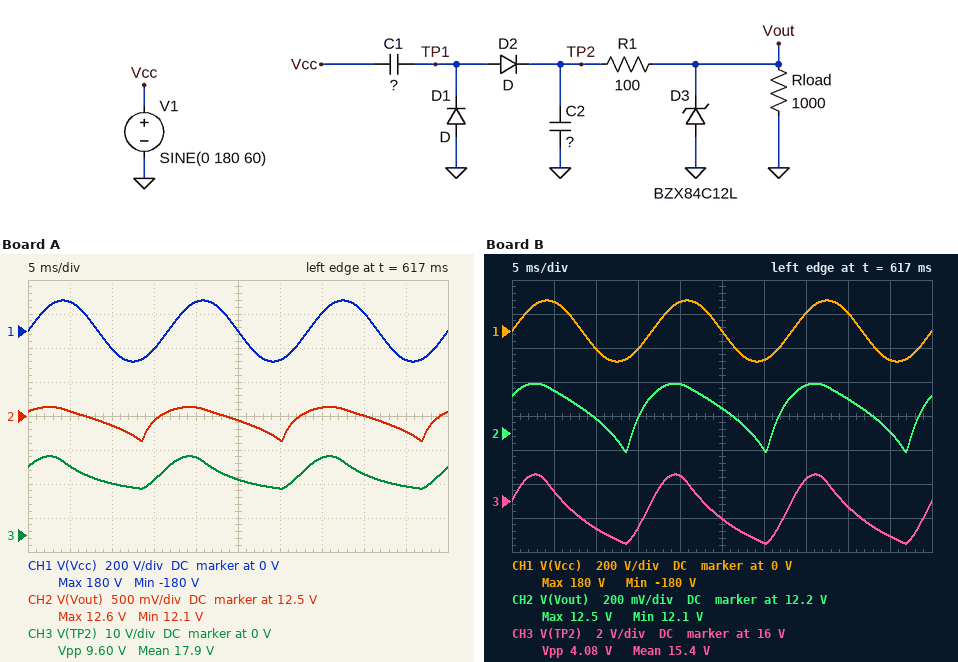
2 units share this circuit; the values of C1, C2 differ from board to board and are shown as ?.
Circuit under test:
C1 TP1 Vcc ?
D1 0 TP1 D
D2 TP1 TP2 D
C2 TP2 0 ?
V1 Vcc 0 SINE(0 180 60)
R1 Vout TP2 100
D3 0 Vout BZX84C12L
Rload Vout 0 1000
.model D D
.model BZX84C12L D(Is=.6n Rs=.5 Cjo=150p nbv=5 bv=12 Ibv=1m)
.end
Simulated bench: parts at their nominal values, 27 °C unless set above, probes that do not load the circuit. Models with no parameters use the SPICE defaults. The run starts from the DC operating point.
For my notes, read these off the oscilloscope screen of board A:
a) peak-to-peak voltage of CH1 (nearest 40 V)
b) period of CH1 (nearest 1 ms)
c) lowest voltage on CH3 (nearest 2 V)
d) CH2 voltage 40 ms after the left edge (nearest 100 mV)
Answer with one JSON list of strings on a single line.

["360 V", "17 ms", "14 V", "12.5 V"]
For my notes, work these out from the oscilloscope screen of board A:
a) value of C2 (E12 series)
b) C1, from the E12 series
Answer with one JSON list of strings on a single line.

["47 µF", "2.7 µF"]
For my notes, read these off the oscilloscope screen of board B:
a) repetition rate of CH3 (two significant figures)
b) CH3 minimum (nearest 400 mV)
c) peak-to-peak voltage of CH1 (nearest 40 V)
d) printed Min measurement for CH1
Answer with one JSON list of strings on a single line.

["60 Hz", "13.6 V", "360 V", "-180 V"]
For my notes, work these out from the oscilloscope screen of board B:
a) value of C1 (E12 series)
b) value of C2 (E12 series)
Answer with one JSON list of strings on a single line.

["1.5 µF", "68 µF"]
